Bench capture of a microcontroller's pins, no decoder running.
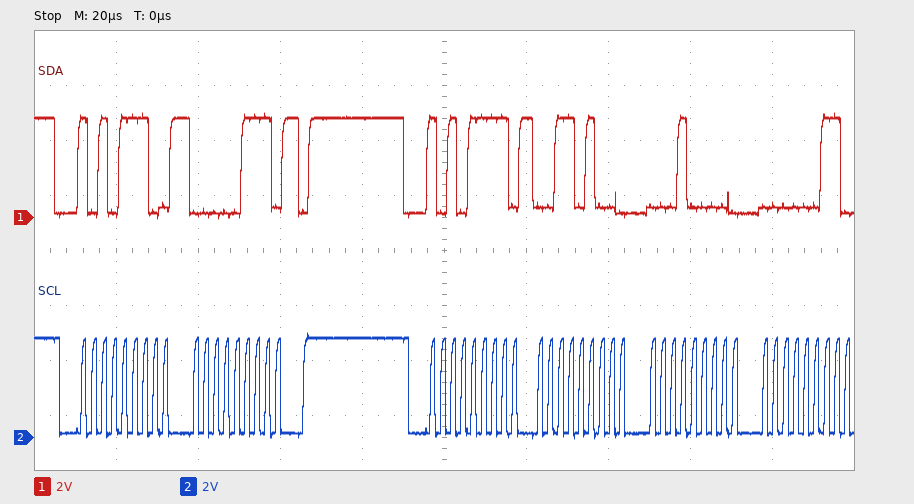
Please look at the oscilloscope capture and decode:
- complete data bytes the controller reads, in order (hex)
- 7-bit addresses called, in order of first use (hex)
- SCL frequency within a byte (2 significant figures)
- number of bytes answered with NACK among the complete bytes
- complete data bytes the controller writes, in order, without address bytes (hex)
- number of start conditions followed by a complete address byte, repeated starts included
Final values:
34 10 03
0x57
400 kHz
0
07
2
